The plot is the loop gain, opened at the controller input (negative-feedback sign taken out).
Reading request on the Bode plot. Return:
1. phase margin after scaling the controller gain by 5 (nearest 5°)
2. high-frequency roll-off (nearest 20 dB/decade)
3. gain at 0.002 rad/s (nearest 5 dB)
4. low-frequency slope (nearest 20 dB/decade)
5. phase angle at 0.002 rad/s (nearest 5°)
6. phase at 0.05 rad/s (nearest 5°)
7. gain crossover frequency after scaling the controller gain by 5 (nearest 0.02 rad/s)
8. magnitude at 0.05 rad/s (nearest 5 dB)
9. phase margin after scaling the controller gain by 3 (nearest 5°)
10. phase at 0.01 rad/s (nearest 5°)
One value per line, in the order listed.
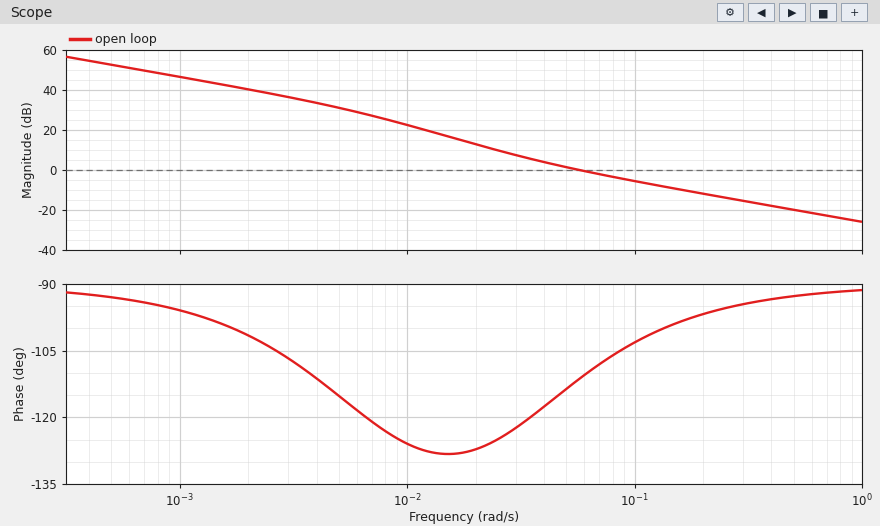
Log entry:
85°
-20 dB/decade
40 dB
-20 dB/decade
-100°
-115°
0.26 rad/s
0 dB
80°
-125°
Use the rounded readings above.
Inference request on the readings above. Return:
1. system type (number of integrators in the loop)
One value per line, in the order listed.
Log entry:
1
